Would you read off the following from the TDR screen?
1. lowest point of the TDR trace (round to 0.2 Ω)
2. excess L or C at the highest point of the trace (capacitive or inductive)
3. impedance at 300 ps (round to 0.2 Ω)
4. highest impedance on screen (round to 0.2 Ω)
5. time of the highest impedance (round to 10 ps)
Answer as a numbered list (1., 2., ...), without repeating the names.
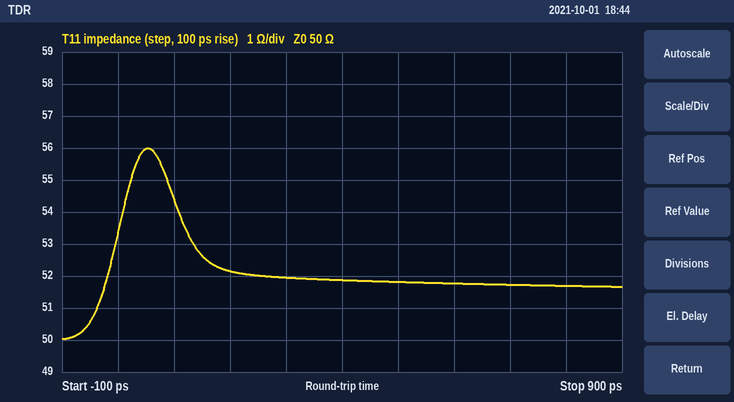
1. 50.0 Ω
2. inductive
3. 52.0 Ω
4. 56.0 Ω
5. 50 ps
